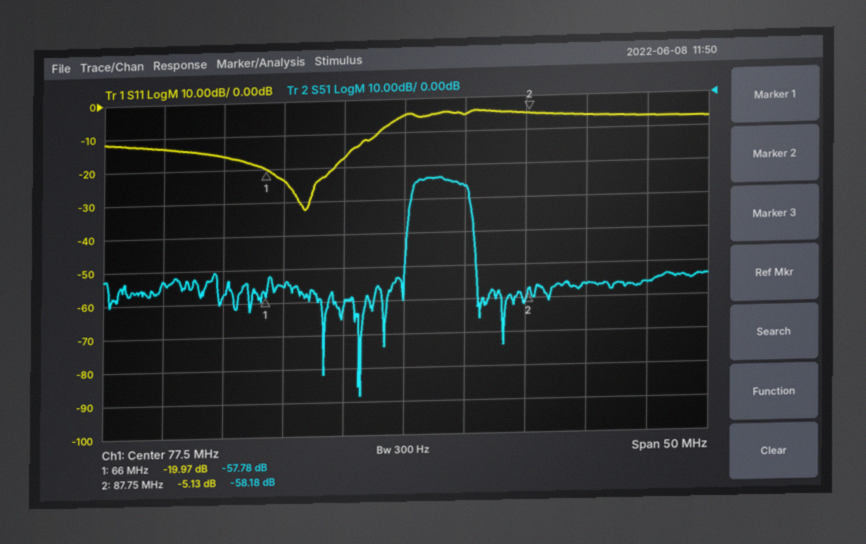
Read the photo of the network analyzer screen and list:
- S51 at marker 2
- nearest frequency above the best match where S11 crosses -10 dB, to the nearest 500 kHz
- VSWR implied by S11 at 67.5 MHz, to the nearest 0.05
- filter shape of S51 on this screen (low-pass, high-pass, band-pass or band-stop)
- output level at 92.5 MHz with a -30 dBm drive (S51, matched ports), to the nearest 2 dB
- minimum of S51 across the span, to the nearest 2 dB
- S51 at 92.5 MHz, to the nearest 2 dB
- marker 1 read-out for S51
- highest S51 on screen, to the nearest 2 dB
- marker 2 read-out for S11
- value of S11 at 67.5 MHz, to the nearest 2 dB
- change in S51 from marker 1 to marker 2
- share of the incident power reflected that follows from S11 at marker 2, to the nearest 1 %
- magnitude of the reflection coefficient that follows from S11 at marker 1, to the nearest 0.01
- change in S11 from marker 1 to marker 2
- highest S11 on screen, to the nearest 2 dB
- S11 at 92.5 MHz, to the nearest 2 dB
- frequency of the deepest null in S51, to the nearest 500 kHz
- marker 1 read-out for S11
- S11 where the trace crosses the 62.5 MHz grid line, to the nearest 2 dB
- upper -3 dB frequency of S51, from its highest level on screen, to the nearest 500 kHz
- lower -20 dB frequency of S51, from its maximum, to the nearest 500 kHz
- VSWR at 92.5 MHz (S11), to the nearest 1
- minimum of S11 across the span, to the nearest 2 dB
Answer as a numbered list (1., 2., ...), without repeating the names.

1. -58.18 dB
2. 75.5 MHz
3. 1.15
4. band-pass
5. -86 dBm
6. -88 dB
7. -56 dB
8. -57.78 dB
9. -24 dB
10. -5.13 dB
11. -24 dB
12. -0.40 dB
13. 31 %
14. 0.10
15. 14.84 dB
16. -4 dB
17. -6 dB
18. 74.0 MHz
19. -19.97 dB
20. -16 dB
21. 82.5 MHz
22. 77.5 MHz
23. 3
24. -32 dB
